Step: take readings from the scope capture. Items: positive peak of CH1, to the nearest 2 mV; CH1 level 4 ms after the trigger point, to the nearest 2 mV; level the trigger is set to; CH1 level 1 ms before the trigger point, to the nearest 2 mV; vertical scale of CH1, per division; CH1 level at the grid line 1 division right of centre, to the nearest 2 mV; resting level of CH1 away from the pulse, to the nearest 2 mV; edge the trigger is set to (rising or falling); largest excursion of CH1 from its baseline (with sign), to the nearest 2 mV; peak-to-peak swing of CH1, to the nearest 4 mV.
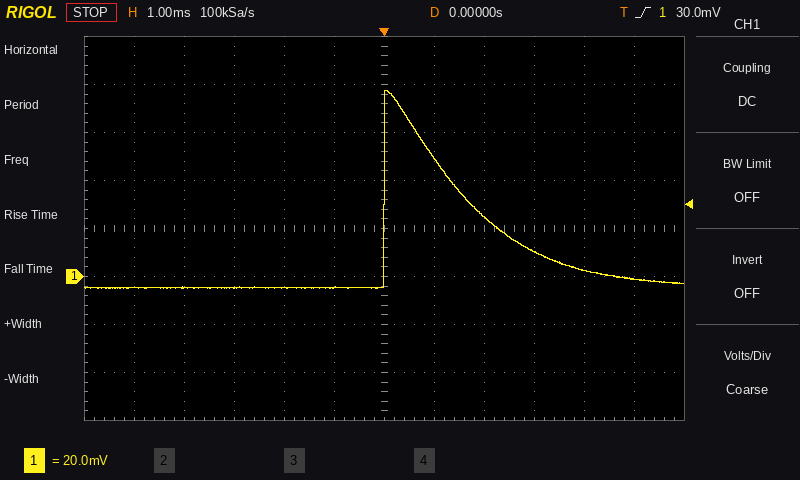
78 mV
2 mV
30.0 mV
-4 mV
20 mV
50 mV
-4 mV
rising
+82 mV
84 mV
